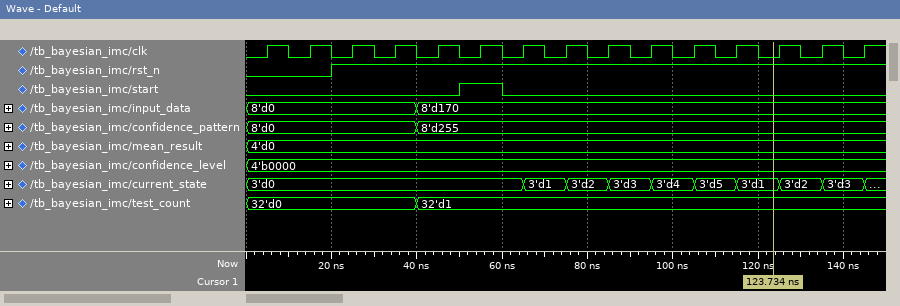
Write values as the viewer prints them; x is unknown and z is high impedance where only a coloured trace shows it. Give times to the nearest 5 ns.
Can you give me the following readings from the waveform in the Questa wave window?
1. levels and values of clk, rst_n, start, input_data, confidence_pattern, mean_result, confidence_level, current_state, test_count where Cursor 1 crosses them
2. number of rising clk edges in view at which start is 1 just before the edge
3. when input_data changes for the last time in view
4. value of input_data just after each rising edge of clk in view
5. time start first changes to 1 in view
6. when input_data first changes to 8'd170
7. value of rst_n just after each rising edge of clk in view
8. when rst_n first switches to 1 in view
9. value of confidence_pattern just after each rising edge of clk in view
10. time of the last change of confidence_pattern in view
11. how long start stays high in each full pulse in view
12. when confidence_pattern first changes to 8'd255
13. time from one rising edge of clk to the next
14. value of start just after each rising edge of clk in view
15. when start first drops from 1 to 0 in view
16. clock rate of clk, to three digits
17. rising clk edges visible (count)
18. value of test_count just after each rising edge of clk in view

clk=0, rst_n=1, start=0, input_data=8'd170, confidence_pattern=8'd255, mean_result=4'd0, confidence_level=4'b0000, current_state=3'd1, test_count=32'd1
1
40 ns
8'd0, 8'd0, 8'd0, 8'd0, 8'd170, 8'd170, 8'd170, 8'd170, 8'd170, 8'd170, 8'd170, 8'd170, 8'd170, 8'd170, 8'd170
50 ns
40 ns
0 0 1 1 1 1 1 1 1 1 1 1 1 1 1
20 ns
8'd0, 8'd0, 8'd0, 8'd0, 8'd255, 8'd255, 8'd255, 8'd255, 8'd255, 8'd255, 8'd255, 8'd255, 8'd255, 8'd255, 8'd255
40 ns
10 ns
40 ns
10 ns
0 0 0 0 0 1 0 0 0 0 0 0 0 0 0
60 ns
100 MHz
15
32'd0, 32'd0, 32'd0, 32'd0, 32'd1, 32'd1, 32'd1, 32'd1, 32'd1, 32'd1, 32'd1, 32'd1, 32'd1, 32'd1, 32'd1
